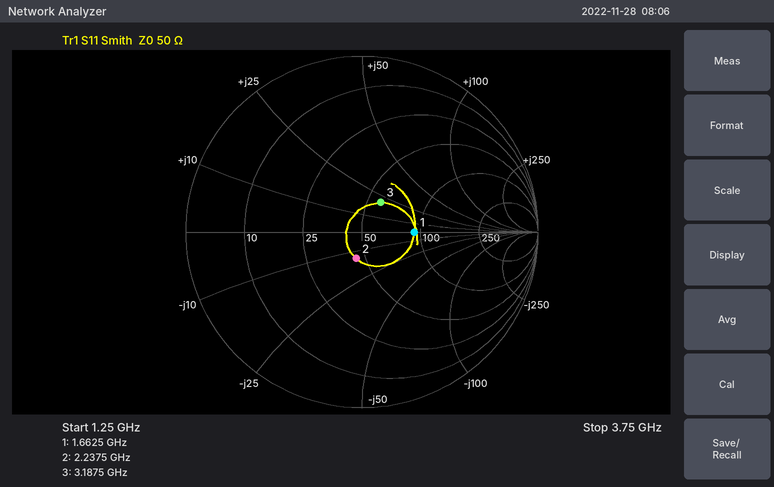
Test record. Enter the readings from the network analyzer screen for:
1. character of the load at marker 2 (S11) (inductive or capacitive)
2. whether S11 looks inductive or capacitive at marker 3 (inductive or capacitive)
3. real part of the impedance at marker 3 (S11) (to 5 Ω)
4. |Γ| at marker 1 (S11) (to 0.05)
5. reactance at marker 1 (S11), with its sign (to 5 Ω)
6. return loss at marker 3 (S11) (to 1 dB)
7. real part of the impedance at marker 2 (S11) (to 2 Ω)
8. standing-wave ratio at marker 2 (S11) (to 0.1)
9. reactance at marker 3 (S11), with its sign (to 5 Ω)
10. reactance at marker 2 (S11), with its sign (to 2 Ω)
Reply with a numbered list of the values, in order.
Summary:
1. capacitive
2. inductive
3. 60 Ω
4. 0.30
5. 0 Ω
6. 14 dB
7. 44 Ω
8. 1.4
9. +20 Ω
10. -14 Ω
